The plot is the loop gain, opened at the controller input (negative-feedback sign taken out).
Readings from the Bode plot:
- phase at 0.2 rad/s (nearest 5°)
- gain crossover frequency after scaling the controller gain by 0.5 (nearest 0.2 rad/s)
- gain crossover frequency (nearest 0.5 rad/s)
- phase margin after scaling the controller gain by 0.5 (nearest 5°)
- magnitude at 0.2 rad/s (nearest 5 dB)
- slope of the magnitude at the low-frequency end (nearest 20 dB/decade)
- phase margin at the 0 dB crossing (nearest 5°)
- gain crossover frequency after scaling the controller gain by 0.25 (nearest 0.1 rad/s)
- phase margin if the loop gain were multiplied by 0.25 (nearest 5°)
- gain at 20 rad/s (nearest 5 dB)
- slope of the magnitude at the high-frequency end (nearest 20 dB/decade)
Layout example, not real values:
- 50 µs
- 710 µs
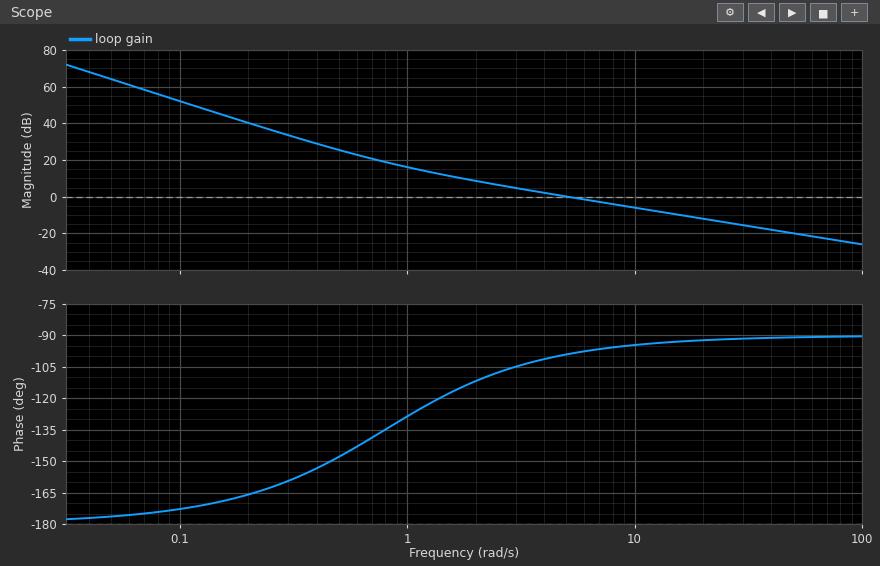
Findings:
- -165°
- 2.6 rad/s
- 5.0 rad/s
- 75°
- 40 dB
- -40 dB/decade
- 80°
- 1.4 rad/s
- 60°
- -10 dB
- -20 dB/decade
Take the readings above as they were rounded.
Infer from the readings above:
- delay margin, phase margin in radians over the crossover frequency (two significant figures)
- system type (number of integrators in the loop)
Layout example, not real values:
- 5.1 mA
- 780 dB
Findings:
- 0.28 s
- 2
